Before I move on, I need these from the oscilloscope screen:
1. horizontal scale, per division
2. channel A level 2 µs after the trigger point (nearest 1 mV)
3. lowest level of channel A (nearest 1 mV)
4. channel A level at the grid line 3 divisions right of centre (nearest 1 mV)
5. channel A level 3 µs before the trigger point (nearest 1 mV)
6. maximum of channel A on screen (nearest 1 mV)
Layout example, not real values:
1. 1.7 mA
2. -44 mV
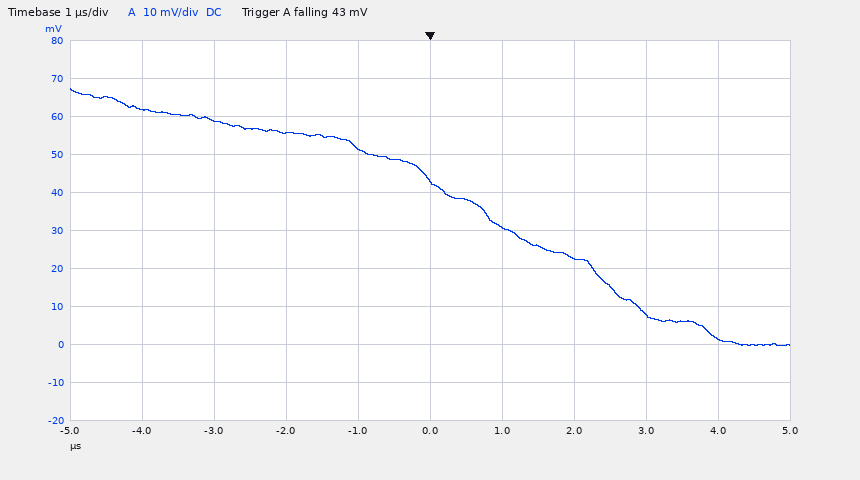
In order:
1. 1 µs
2. 23 mV
3. 0 mV
4. 8 mV
5. 59 mV
6. 67 mV
